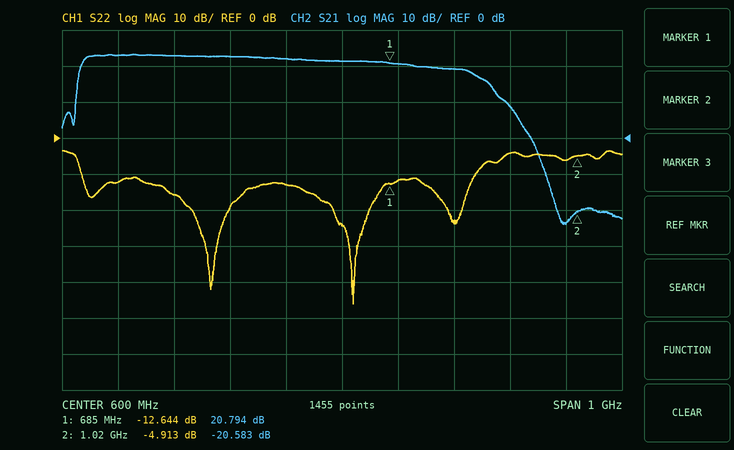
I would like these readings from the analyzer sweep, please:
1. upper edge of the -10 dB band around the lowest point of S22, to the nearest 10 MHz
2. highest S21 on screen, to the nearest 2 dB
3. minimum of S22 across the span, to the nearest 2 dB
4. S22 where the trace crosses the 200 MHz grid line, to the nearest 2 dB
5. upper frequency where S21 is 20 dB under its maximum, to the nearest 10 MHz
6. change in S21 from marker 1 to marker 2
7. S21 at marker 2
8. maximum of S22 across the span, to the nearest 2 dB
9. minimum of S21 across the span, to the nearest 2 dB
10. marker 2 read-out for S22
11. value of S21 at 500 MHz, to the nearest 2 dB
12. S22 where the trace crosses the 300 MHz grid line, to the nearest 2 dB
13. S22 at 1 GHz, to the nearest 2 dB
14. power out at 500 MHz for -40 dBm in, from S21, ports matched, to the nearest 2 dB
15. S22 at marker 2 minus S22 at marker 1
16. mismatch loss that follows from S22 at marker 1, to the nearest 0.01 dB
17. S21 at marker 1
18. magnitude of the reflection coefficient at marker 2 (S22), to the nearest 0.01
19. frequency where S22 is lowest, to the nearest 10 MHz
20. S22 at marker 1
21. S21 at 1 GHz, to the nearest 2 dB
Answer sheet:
840 MHz
24 dB
-46 dB
-12 dB
920 MHz
-41.377 dB
-20.583 dB
-4 dB
-24 dB
-4.913 dB
22 dB
-16 dB
-6 dB
-18 dBm
7.731 dB
0.24 dB
20.794 dB
0.57
620 MHz
-12.644 dB
-24 dB
